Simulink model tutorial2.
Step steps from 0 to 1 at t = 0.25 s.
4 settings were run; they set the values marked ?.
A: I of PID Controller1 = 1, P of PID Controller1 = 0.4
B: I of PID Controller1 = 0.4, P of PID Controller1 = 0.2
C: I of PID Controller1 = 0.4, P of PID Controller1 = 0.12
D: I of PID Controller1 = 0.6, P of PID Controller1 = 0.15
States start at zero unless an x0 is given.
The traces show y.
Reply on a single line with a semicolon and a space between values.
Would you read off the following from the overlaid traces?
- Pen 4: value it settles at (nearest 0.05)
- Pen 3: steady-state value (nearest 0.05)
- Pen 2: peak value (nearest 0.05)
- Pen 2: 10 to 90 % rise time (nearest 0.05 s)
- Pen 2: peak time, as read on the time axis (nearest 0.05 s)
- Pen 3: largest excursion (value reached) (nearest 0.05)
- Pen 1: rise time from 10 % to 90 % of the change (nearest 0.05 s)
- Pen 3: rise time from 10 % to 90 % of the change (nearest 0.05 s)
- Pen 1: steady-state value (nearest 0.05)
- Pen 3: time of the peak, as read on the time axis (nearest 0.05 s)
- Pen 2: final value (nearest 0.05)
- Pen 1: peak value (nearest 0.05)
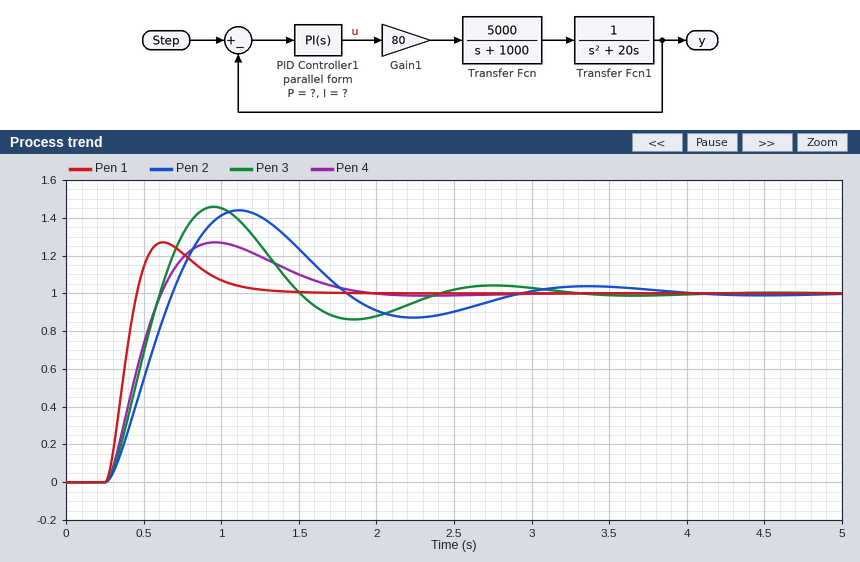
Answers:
1.00; 1.00; 1.45; 0.30 s; 1.10 s; 1.45; 0.15 s; 0.25 s; 1.00; 0.95 s; 1.00; 1.25
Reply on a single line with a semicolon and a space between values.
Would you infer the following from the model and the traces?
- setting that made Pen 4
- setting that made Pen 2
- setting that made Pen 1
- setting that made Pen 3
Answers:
B; C; A; D
